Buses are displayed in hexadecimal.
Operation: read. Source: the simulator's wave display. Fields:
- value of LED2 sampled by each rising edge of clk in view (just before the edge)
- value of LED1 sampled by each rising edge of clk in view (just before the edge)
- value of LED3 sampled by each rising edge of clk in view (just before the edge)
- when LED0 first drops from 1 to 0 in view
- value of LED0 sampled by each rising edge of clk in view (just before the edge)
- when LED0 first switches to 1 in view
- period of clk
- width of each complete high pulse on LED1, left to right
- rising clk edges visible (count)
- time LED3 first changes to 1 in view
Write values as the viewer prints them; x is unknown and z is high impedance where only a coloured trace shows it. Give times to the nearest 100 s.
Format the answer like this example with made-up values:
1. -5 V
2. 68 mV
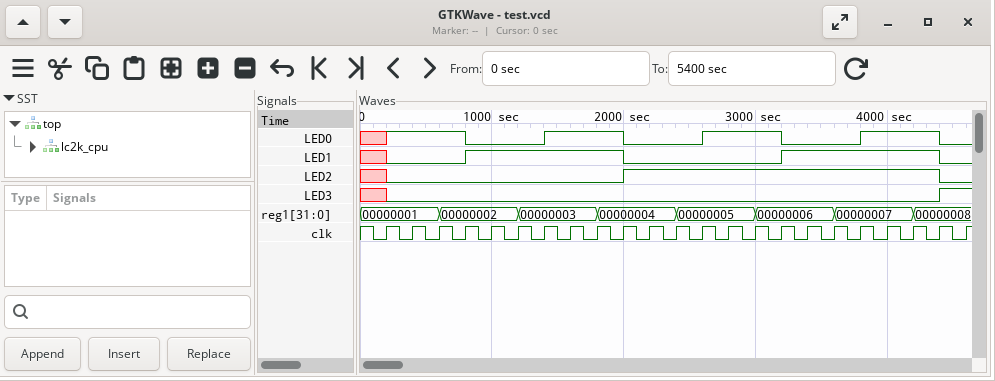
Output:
1. x 0 0 0 0 0 0 0 0 0 1 1 1 1 1 1 1 1 1 1 1 1 0
2. x 0 0 0 1 1 1 1 1 1 0 0 0 0 0 0 1 1 1 1 1 1 0
3. x 0 0 0 0 0 0 0 0 0 0 0 0 0 0 0 0 0 0 0 0 0 1
4. 800 s
5. x 1 1 1 0 0 0 1 1 1 0 0 0 1 1 1 0 0 0 1 1 1 0
6. 200 s
7. 200 s
8. 1200 s, 1200 s
9. 23
10. 4400 s
